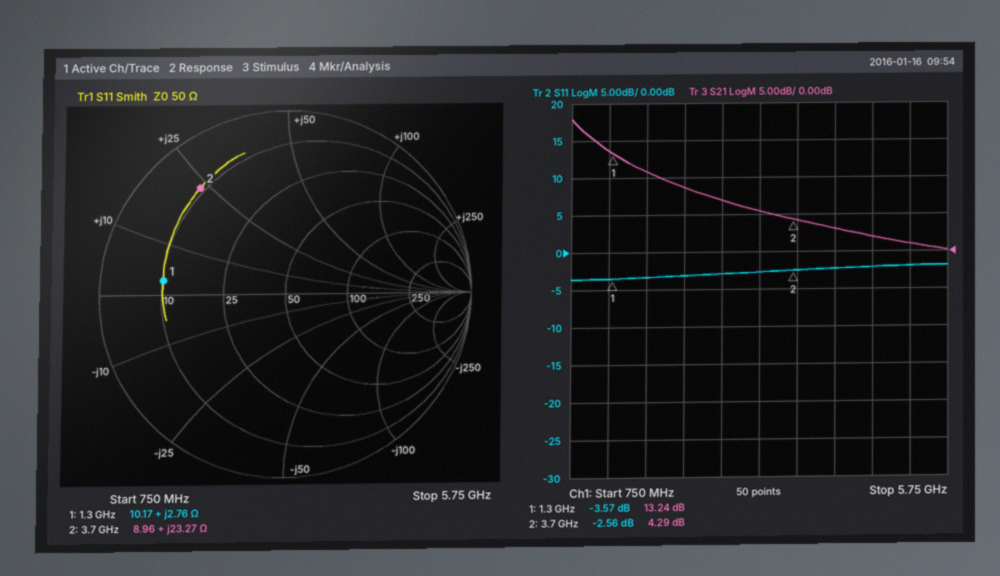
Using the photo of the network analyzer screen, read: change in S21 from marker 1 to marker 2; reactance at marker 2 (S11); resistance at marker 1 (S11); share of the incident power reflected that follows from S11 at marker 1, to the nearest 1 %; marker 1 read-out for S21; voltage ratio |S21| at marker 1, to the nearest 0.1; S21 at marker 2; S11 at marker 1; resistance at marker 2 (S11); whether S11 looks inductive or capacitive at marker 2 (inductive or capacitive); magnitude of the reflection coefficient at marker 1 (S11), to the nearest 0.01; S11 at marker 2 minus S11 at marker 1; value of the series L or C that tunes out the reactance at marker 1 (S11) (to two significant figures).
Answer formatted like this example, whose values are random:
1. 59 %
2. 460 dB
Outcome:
1. -8.95 dB
2. +23.27 Ω
3. 10.17 Ω
4. 44 %
5. 13.24 dB
6. 4.6
7. 4.29 dB
8. -3.57 dB
9. 8.96 Ω
10. inductive
11. 0.66
12. 1.01 dB
13. 44 pF
